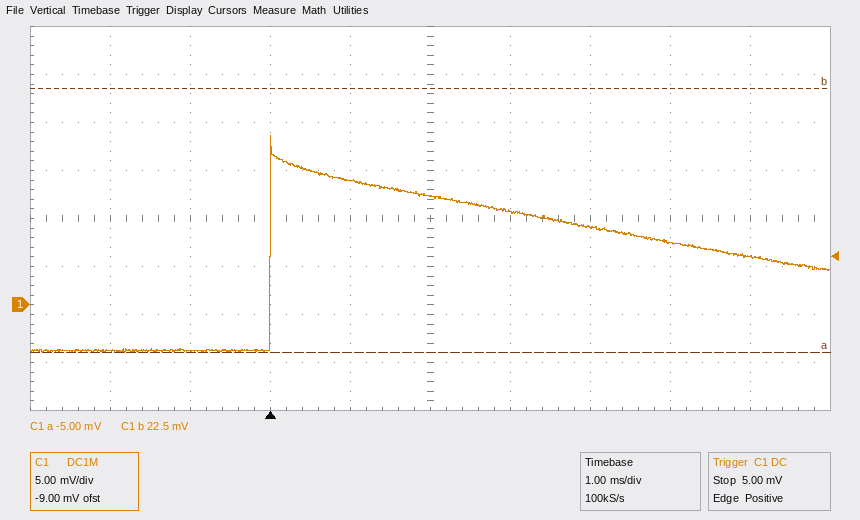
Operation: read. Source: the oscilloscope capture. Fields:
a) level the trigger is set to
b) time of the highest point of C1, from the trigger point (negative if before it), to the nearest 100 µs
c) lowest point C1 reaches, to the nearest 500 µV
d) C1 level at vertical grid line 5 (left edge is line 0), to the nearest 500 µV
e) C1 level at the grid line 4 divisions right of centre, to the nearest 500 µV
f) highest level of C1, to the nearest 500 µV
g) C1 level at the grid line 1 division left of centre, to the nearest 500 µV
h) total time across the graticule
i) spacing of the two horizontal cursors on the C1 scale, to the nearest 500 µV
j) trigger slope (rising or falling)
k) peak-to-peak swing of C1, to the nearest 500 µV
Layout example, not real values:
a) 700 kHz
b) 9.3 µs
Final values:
a) 5.00 mV
b) 0.0 ms
c) -5.0 mV
d) 11.5 mV
e) 5.0 mV
f) 17.5 mV
g) 13.0 mV
h) 10 ms
i) 27.5 mV
j) rising
k) 22.5 mV
